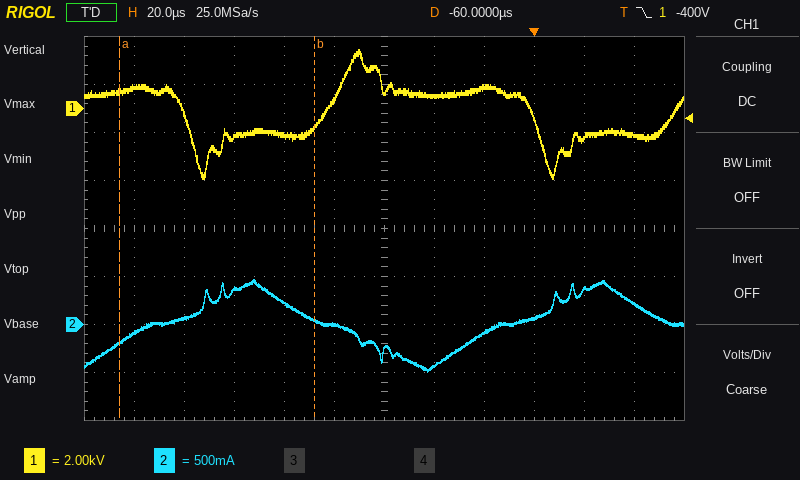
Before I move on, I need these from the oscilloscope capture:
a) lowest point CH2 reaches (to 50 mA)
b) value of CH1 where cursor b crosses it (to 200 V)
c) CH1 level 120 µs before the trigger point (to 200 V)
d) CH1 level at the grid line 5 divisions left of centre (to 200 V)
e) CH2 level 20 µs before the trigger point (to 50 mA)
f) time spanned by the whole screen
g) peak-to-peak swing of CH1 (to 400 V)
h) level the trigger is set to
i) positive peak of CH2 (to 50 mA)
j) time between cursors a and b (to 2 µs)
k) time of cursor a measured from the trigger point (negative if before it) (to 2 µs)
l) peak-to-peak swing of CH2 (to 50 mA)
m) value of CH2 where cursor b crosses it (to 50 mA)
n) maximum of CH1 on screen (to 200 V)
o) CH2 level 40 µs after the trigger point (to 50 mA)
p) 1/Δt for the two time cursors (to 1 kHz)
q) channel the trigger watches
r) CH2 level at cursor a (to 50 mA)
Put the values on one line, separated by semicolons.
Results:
-500 mA; -800 V; -1.2 kV; 800 V; -100 mA; 240 µs; 5.2 kV; -400 V; 450 mA; 78 µs; -166 µs; 950 mA; 50 mA; 2.4 kV; 200 mA; 13 kHz; CH1; -200 mA
